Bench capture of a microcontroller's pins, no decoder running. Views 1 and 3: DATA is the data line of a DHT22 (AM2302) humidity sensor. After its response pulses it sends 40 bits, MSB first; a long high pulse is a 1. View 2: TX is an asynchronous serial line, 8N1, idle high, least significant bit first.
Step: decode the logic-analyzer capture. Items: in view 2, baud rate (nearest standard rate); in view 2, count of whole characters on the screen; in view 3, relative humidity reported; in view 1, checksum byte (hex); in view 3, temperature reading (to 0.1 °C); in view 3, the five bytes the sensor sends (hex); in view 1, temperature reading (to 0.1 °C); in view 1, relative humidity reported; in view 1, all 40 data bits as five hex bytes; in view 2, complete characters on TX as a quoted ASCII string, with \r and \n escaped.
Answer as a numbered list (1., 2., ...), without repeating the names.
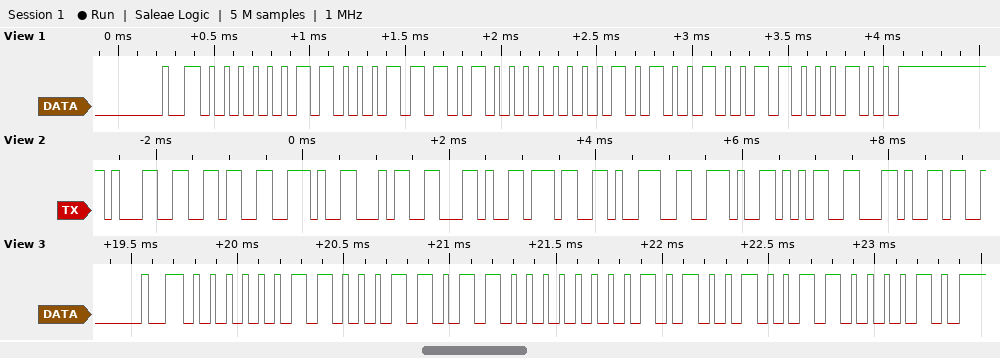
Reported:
1. 9600 baud
2. 10
3. 79.5 %
4. 0xC4
5. 16.4 °C
6. 03 1B 00 A4 C2
7. 16.4 °C
8. 79.7 %
9. 03 1D 00 A4 C4
10. "16.4,79.5,"
